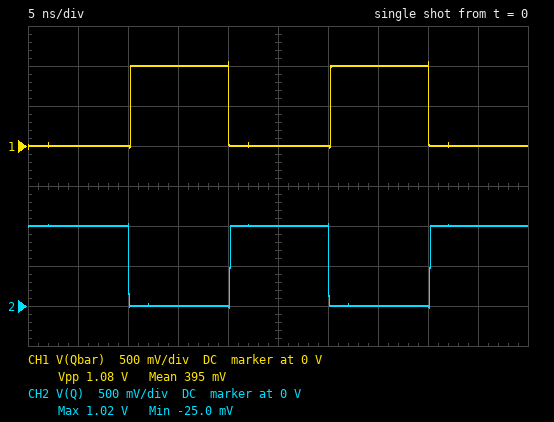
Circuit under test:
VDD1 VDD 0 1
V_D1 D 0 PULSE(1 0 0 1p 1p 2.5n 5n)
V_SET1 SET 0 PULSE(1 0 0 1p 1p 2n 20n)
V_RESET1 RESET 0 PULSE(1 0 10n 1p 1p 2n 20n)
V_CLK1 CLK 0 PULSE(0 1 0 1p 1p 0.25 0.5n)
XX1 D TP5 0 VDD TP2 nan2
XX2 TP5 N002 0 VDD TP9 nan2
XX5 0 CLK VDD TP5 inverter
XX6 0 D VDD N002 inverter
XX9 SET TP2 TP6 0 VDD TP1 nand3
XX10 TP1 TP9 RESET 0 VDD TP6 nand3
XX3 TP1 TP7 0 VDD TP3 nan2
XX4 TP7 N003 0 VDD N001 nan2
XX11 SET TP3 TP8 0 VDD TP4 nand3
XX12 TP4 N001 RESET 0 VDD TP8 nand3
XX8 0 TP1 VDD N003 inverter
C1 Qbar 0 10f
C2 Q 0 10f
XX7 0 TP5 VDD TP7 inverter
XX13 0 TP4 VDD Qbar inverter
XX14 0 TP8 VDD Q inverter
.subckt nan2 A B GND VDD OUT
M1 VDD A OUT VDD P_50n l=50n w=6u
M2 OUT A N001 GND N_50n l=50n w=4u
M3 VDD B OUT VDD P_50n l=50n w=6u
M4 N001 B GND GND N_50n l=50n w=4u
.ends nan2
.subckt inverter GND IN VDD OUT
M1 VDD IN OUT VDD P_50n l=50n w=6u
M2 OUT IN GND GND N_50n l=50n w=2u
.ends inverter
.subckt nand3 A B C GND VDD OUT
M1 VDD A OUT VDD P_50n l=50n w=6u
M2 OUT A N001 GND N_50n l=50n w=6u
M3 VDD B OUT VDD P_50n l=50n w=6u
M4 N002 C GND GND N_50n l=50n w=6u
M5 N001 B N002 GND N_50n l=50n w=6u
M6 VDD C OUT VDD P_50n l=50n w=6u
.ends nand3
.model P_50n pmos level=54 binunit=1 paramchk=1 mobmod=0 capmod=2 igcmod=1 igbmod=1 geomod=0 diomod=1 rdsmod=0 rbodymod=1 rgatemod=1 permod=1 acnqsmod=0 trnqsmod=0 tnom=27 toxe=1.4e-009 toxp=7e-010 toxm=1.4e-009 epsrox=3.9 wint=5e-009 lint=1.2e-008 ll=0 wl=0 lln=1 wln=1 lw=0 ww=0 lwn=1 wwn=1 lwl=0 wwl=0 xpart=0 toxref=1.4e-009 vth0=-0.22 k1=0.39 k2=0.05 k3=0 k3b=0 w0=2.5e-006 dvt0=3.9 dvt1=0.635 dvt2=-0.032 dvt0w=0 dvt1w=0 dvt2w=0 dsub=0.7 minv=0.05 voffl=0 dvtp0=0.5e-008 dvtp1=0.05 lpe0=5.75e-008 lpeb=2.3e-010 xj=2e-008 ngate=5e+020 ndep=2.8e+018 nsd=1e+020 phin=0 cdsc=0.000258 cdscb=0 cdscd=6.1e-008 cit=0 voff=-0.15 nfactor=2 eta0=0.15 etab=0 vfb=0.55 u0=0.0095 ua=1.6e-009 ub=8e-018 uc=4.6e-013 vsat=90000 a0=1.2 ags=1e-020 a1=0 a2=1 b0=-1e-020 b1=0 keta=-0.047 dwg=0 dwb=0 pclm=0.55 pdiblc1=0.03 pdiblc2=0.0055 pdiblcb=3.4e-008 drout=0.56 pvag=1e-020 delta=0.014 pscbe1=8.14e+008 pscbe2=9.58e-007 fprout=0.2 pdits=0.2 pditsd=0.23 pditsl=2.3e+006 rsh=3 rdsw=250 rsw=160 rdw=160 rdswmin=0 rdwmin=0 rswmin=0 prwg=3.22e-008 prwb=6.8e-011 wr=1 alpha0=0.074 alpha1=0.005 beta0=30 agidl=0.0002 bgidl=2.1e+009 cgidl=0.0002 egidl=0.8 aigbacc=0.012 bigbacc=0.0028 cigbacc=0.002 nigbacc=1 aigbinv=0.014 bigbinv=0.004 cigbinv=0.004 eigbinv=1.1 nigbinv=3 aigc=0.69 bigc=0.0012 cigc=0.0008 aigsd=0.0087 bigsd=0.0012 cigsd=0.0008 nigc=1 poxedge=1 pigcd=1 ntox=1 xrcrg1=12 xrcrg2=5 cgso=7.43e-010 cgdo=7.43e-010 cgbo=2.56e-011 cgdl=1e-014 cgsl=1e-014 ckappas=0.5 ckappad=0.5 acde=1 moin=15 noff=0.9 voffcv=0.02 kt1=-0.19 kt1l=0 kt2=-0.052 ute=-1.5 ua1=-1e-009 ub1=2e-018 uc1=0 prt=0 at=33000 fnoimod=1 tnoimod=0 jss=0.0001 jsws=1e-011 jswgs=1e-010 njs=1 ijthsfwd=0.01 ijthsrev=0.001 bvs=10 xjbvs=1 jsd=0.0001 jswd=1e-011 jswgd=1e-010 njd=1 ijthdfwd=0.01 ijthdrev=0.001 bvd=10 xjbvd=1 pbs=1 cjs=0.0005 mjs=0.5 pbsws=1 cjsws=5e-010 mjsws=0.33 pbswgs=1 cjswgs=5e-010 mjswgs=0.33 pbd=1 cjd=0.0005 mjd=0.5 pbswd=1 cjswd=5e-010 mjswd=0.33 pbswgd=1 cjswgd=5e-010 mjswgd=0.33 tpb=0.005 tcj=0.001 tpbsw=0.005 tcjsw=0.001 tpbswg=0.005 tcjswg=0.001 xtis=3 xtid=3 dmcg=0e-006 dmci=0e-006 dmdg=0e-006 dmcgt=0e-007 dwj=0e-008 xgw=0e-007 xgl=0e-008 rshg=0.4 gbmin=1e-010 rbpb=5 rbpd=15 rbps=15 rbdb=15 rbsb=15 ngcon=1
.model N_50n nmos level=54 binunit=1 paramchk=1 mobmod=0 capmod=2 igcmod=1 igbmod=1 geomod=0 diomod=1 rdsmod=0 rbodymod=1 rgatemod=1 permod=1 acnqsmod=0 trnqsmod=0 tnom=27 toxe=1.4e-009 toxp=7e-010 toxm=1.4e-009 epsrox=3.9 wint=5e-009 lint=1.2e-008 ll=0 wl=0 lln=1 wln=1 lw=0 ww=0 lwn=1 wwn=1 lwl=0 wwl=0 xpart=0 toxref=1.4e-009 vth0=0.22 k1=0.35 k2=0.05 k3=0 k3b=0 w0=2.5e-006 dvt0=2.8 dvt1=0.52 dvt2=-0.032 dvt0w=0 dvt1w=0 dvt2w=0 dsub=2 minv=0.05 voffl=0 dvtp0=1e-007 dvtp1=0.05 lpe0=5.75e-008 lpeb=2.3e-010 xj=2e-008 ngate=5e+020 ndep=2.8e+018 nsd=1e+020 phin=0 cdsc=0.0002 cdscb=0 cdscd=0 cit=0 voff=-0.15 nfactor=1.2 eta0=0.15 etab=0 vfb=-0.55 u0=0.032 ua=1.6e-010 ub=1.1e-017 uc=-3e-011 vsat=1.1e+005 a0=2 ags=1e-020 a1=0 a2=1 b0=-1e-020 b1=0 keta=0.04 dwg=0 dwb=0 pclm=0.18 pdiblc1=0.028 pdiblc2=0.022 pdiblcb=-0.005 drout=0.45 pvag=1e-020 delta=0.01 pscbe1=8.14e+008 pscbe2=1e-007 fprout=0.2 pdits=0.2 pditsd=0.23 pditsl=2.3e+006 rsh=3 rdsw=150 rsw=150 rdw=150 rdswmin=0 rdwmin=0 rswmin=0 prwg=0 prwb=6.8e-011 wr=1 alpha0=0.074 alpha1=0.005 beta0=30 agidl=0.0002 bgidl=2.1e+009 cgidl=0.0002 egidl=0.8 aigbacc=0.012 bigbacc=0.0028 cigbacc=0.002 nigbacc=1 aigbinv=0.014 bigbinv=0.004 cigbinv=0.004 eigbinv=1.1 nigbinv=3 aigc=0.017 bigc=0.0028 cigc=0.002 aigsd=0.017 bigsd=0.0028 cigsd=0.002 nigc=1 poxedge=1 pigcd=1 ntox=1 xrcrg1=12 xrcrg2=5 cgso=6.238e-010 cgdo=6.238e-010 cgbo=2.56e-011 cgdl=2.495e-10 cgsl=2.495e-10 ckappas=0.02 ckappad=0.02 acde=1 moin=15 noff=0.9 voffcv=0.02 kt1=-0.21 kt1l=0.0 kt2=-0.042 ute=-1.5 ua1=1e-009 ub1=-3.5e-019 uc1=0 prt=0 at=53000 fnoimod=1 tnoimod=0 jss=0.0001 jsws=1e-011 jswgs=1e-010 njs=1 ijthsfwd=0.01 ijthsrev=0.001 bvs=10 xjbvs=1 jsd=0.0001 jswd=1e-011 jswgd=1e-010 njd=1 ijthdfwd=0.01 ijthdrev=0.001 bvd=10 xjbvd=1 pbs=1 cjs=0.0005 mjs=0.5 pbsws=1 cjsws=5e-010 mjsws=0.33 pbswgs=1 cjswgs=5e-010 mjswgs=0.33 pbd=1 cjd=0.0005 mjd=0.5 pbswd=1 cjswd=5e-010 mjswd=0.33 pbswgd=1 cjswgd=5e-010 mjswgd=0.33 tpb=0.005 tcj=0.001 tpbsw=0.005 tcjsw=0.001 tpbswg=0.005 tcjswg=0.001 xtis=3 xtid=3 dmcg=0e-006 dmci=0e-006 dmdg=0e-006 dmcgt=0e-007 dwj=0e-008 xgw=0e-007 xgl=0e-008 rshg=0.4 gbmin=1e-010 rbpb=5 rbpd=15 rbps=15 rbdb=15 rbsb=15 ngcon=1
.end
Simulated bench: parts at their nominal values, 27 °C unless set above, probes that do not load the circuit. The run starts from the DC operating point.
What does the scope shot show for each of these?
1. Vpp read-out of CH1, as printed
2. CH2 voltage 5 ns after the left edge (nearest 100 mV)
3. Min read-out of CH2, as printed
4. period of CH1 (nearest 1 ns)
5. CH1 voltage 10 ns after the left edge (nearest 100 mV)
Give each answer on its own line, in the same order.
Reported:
1.08 V
1.0 V
-25.0 mV
20 ns
0 V
